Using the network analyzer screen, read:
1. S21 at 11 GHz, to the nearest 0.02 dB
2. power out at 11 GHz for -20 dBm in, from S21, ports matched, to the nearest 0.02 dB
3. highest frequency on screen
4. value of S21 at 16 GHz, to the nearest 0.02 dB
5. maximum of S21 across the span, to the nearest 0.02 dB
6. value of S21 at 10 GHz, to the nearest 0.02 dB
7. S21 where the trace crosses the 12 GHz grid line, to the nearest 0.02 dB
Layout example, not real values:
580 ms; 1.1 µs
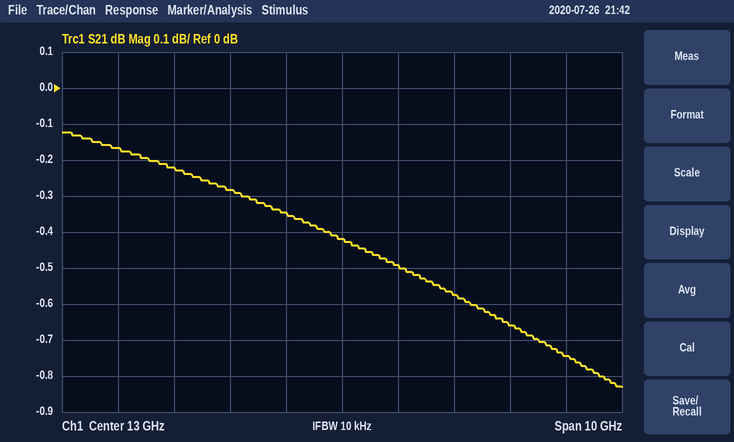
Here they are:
-0.28 dB; -20.28 dBm; 18 GHz; -0.66 dB; -0.12 dB; -0.22 dB; -0.34 dB
